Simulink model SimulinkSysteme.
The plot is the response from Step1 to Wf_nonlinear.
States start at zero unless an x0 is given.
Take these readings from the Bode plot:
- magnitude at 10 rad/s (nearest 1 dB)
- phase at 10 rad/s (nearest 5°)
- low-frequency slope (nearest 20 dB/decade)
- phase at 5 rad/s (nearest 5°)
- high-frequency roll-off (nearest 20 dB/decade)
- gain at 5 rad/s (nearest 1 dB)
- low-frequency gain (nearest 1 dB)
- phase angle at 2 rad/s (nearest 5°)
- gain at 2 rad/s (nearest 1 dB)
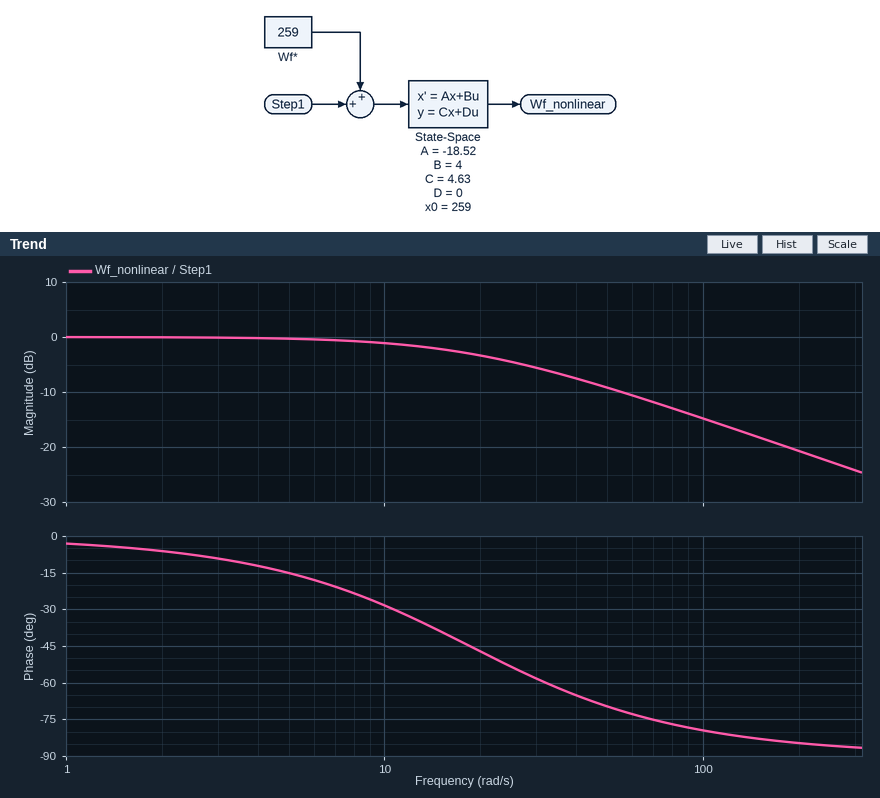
-1 dB
-30°
0 dB/decade
-15°
-20 dB/decade
0 dB
0 dB
-5°
0 dB
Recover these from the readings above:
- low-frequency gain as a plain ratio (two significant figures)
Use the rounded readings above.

1.0
